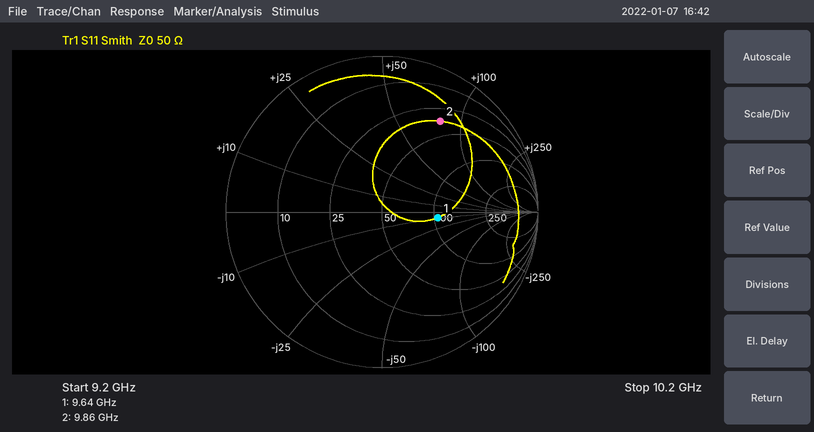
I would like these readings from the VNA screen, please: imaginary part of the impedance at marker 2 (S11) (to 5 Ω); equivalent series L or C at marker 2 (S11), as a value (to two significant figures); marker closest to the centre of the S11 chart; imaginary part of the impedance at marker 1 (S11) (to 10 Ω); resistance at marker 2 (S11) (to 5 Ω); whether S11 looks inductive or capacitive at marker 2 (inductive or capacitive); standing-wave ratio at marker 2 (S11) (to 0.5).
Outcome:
+80 Ω
1.3 nH
marker 1
-10 Ω
35 Ω
inductive
5.5
